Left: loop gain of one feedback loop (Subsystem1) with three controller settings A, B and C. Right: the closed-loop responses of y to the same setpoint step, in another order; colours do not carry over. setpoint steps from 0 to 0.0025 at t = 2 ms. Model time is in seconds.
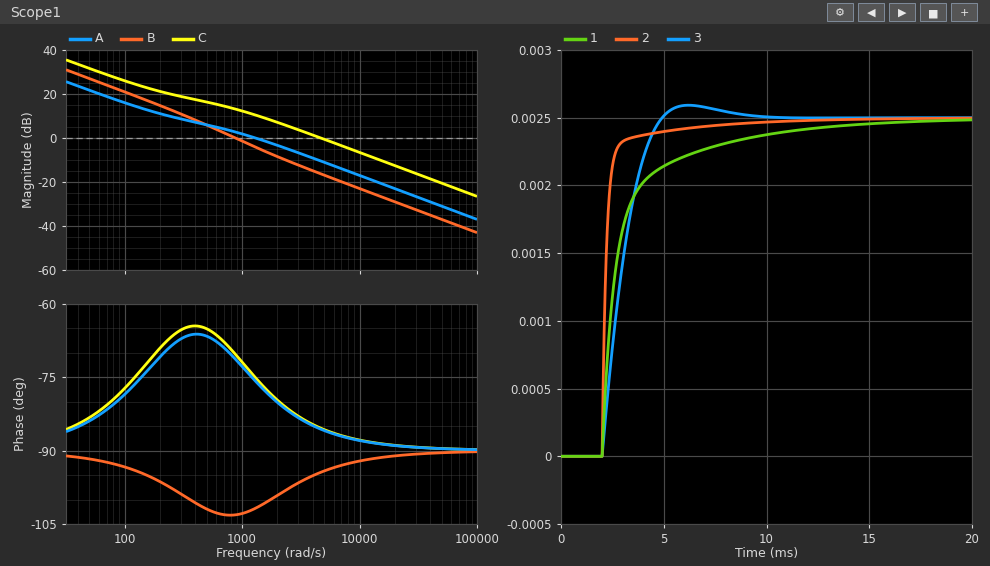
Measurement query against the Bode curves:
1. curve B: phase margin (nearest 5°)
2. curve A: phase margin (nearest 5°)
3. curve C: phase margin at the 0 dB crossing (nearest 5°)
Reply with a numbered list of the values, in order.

1. 75°
2. 105°
3. 95°
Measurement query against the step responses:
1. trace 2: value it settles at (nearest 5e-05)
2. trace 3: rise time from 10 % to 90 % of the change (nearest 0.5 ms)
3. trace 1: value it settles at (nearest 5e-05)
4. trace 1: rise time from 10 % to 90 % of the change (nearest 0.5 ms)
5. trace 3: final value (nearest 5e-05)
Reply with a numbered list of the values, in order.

1. 0.00250
2. 2.0 ms
3. 0.00250
4. 4.5 ms
5. 0.00250
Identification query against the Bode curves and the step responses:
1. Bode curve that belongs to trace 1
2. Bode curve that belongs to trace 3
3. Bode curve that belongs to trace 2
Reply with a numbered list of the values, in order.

1. A
2. B
3. C
